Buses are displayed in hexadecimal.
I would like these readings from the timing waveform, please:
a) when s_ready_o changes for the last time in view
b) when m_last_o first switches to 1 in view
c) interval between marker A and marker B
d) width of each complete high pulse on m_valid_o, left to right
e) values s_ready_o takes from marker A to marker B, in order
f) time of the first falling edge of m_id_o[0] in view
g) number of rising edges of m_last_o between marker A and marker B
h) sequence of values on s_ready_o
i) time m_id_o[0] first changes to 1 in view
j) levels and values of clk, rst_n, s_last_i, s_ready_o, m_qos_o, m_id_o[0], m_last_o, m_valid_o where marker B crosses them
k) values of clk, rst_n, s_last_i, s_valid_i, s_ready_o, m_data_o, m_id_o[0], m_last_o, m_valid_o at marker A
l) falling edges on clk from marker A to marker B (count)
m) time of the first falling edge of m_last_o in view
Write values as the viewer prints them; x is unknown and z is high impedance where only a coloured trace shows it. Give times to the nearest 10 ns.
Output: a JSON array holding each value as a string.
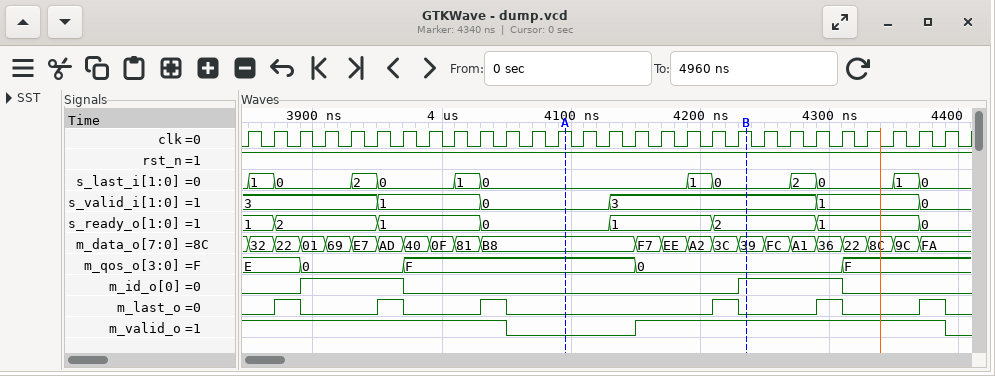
["4370 ns", "3870 ns", "140 ns", "240 ns", "0, 1, 2", "3970 ns", "1", "1, 2, 1, 0, 1, 2, 1, 0", "3890 ns", "clk=1, rst_n=1, s_last_i=0, s_ready_o=2, m_qos_o=0, m_id_o[0]=1, m_last_o=0, m_valid_o=1", "clk=1, rst_n=1, s_last_i=0, s_valid_i=0, s_ready_o=0, m_data_o=B8, m_id_o[0]=0, m_last_o=0, m_valid_o=0", "7", "3890 ns"]
